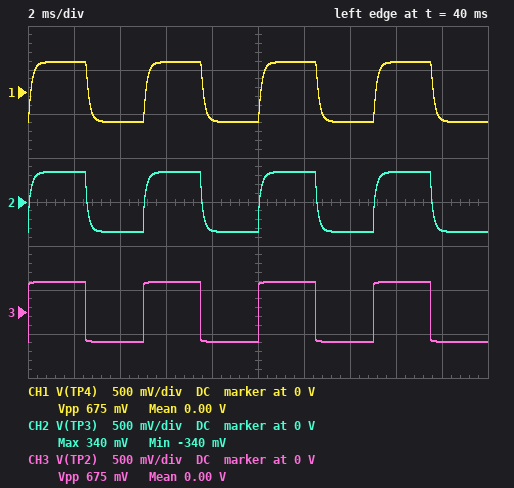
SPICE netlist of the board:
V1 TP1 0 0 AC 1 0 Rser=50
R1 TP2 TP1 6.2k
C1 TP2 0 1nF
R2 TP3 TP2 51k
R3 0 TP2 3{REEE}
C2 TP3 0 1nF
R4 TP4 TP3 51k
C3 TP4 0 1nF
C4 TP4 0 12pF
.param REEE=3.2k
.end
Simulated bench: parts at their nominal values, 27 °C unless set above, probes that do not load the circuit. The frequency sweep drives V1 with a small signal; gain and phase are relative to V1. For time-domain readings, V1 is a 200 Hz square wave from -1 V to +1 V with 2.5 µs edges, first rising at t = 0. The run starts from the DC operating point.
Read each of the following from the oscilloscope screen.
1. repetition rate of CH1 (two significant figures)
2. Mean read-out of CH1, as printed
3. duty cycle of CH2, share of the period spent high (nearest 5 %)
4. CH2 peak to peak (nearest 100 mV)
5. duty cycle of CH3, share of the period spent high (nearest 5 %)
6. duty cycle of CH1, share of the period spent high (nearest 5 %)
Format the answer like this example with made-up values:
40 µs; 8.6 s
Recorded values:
200 Hz; 0.00 V; 50 %; 700 mV; 50 %; 50 %
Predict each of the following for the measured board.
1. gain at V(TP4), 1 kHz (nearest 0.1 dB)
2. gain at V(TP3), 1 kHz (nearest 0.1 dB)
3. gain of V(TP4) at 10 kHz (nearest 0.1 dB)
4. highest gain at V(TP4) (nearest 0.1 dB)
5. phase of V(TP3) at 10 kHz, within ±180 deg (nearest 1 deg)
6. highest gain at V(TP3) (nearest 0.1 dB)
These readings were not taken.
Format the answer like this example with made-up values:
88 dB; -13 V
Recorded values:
-11.9 dB; -11.5 dB; -32.4 dB; -9.4 dB; -69 deg; -9.4 dB
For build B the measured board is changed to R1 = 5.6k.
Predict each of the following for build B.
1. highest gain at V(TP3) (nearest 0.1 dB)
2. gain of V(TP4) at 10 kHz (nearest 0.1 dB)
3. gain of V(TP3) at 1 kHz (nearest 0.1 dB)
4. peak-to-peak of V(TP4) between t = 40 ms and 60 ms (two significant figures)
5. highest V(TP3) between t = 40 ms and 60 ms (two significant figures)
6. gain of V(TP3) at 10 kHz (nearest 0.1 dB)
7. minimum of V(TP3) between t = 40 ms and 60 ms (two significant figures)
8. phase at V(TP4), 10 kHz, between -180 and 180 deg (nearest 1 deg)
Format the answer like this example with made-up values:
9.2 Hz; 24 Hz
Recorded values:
-8.8 dB; -31.8 dB; -10.9 dB; 720 mV; 360 mV; -21.2 dB; -360 mV; -142 deg
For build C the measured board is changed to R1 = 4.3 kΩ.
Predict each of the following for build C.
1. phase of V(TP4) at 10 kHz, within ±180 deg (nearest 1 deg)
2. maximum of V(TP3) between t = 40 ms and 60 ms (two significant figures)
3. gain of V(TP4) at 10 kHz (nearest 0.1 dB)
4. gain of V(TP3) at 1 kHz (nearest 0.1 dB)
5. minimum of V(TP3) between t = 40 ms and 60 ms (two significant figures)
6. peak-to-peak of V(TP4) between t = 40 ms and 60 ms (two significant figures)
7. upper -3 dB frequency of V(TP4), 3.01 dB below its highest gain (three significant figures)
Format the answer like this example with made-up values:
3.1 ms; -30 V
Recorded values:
-141 deg; 420 mV; -30.4 dB; -9.5 dB; -420 mV; 850 mV; 1.13 kHz
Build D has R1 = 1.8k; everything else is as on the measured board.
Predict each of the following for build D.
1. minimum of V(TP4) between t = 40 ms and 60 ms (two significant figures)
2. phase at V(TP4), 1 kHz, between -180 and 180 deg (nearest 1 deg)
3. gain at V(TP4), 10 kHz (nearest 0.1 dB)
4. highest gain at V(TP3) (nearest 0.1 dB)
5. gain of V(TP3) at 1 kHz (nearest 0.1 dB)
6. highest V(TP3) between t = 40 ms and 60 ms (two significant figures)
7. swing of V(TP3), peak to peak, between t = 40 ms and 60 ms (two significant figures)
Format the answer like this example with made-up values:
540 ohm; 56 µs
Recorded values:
-630 mV; -48 deg; -26.8 dB; -4.0 dB; -6.0 dB; 630 mV; 1.3 V
